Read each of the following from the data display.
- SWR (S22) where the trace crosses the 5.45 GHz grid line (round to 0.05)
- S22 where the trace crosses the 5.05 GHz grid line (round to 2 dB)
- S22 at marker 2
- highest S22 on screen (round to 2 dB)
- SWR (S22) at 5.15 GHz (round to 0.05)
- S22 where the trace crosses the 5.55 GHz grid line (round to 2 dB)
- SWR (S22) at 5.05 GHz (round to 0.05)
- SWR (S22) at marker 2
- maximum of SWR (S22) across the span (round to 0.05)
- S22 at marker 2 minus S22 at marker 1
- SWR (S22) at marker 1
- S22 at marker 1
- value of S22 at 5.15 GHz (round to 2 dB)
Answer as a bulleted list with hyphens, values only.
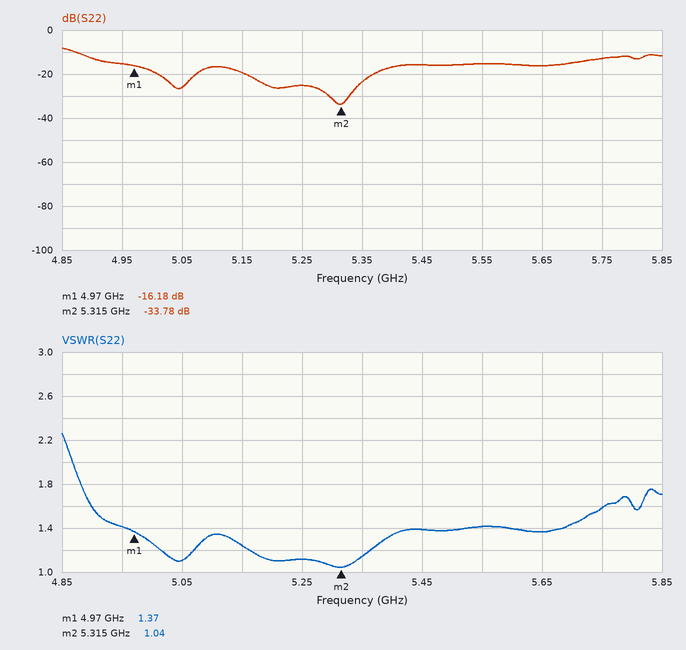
- 1.40
- -26 dB
- -33.78 dB
- -8 dB
- 1.25
- -16 dB
- 1.10
- 1.04
- 2.25
- -17.60 dB
- 1.37
- -16.18 dB
- -20 dB
